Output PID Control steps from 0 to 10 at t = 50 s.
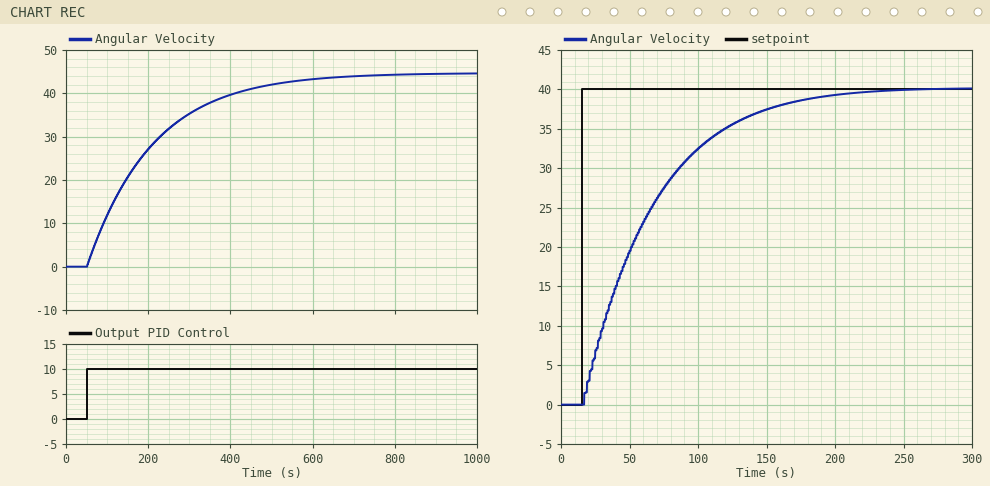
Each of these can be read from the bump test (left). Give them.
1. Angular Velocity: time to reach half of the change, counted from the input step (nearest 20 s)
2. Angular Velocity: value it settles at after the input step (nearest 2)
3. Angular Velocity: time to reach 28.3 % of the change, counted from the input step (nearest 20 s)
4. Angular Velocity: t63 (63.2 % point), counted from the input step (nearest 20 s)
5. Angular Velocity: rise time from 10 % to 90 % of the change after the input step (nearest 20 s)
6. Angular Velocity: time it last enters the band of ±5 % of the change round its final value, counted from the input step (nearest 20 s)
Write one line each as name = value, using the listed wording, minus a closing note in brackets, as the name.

Angular Velocity: time to reach half of the change, counted from the input step = 120 s
Angular Velocity: value it settles at after the input step = 44
Angular Velocity: time to reach 28.3 % of the change, counted from the input step = 60 s
Angular Velocity: t63 (63.2 % point), counted from the input step = 160 s
Angular Velocity: rise time from 10 % to 90 % of the change after the input step = 360 s
Angular Velocity: time it last enters the band of ±5 % of the change round its final value, counted from the input step = 480 s
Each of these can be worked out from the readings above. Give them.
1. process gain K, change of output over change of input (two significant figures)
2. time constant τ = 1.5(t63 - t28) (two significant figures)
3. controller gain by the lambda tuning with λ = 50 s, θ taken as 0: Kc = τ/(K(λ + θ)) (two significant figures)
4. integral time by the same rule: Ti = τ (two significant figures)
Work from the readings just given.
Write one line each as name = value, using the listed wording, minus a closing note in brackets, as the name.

process gain K, change of output over change of input = 4.4
time constant τ = 1.5(t63 - t28) = 150 s
controller gain by the lambda tuning with λ = 50 s, θ taken as 0: Kc = τ/(K(λ + θ)) = 0.68
integral time by the same rule: Ti = τ = 150 s
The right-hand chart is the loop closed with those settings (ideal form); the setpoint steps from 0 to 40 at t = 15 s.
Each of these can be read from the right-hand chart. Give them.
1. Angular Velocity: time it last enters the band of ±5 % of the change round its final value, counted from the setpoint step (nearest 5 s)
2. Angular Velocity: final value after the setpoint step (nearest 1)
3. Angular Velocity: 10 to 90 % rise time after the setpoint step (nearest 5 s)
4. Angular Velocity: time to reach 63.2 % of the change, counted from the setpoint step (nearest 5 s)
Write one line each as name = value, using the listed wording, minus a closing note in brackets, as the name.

Angular Velocity: time it last enters the band of ±5 % of the change round its final value, counted from the setpoint step = 145 s
Angular Velocity: final value after the setpoint step = 40
Angular Velocity: 10 to 90 % rise time after the setpoint step = 110 s
Angular Velocity: time to reach 63.2 % of the change, counted from the setpoint step = 50 s
